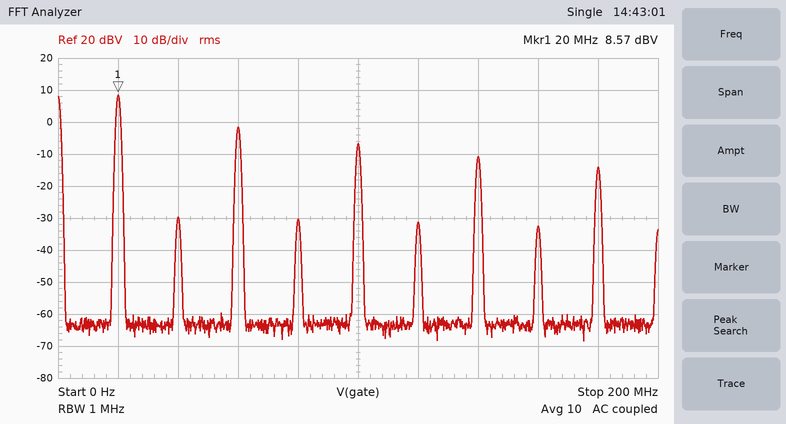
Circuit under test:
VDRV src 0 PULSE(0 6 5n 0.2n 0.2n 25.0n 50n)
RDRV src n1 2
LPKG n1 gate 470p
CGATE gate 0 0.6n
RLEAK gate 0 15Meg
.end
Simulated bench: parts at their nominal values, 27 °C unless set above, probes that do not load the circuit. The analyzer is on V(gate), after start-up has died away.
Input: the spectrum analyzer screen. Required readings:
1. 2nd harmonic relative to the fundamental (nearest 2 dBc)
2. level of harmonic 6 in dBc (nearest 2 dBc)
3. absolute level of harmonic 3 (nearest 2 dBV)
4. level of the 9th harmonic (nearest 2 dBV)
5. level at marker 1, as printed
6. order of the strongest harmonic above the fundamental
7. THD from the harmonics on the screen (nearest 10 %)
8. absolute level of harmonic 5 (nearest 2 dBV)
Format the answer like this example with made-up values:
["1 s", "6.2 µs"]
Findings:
["-38 dBc", "-40 dBc", "-2 dBV", "-14 dBV", "8.57 dBV", "3", "40 %", "-6 dBV"]
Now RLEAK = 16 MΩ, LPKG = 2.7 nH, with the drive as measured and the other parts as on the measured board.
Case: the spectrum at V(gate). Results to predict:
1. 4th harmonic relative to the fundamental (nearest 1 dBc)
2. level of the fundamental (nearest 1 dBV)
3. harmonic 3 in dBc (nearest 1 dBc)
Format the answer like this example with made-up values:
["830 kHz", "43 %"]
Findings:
["-37 dBc", "9 dBV", "-9 dBc"]
